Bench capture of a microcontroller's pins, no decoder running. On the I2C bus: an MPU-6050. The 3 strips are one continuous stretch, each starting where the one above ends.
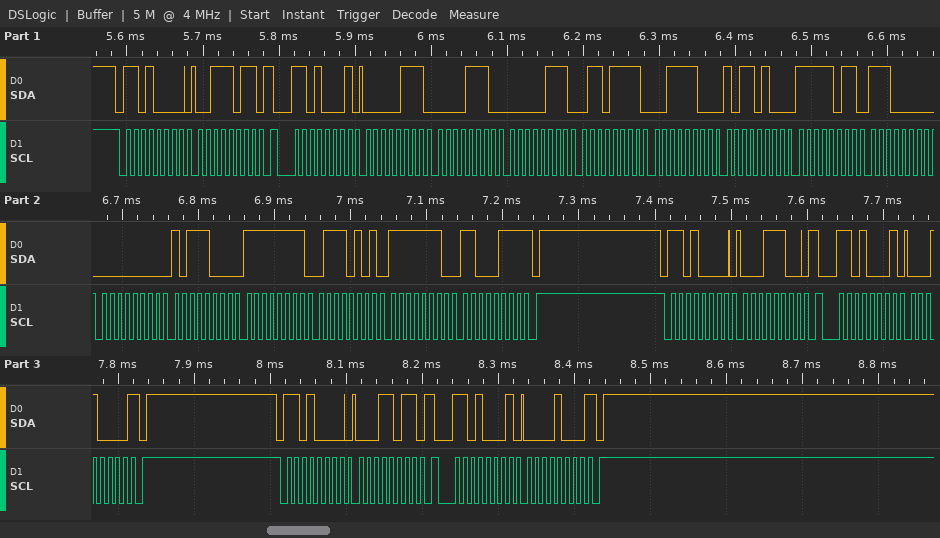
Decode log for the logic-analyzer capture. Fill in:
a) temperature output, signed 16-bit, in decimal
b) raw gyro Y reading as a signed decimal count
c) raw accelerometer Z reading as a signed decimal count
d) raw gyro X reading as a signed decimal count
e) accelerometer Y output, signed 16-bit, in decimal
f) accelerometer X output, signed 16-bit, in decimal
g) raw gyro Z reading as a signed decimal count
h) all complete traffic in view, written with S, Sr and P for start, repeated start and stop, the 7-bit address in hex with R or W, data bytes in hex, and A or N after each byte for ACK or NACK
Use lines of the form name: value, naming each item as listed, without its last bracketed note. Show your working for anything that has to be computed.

temperature output, signed 16-bit, in decimal: 0xFBE0 = -1056
raw gyro Y reading as a signed decimal count: 0xFF75 = -139
raw accelerometer Z reading as a signed decimal count: 0x3CB4 = 15540
raw gyro X reading as a signed decimal count: 0x00B8 = 184
accelerometer Y output, signed 16-bit, in decimal: 0x076F = 1903
accelerometer X output, signed 16-bit, in decimal: 0x070E = 1806
raw gyro Z reading as a signed decimal count: 0xFEC7 = -313
all complete traffic in view, written with S, Sr and P for start, repeated start and stop, the 7-bit address in hex with R or W, data bytes in hex, and A or N after each byte for ACK or NACK: S 68W A 3B A Sr 68R A 07 A 0E A 07 A 6F A 3C A B4 A FB A E0 A 00 A B8 A FF A 75 A FE A C7 N P S 68W A 1C A Sr 68R A 10 N P S 68W A 1B A Sr 68R A 08 N P
